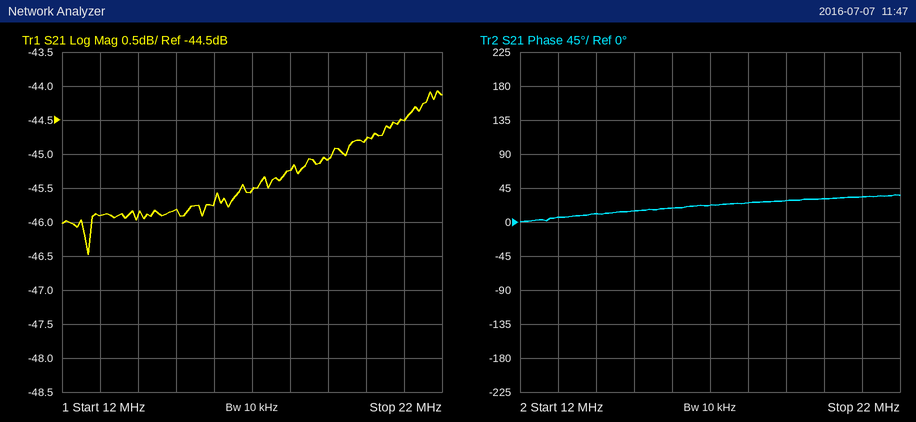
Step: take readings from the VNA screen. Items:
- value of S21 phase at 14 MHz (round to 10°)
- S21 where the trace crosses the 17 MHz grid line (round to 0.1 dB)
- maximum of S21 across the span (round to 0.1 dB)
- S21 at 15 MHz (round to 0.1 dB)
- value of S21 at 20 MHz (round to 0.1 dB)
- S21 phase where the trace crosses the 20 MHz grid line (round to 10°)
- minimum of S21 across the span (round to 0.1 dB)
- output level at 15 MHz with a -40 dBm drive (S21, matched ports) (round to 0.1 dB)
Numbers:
10°
-45.5 dB
-44.1 dB
-45.8 dB
-44.8 dB
30°
-46.5 dB
-85.8 dBm
